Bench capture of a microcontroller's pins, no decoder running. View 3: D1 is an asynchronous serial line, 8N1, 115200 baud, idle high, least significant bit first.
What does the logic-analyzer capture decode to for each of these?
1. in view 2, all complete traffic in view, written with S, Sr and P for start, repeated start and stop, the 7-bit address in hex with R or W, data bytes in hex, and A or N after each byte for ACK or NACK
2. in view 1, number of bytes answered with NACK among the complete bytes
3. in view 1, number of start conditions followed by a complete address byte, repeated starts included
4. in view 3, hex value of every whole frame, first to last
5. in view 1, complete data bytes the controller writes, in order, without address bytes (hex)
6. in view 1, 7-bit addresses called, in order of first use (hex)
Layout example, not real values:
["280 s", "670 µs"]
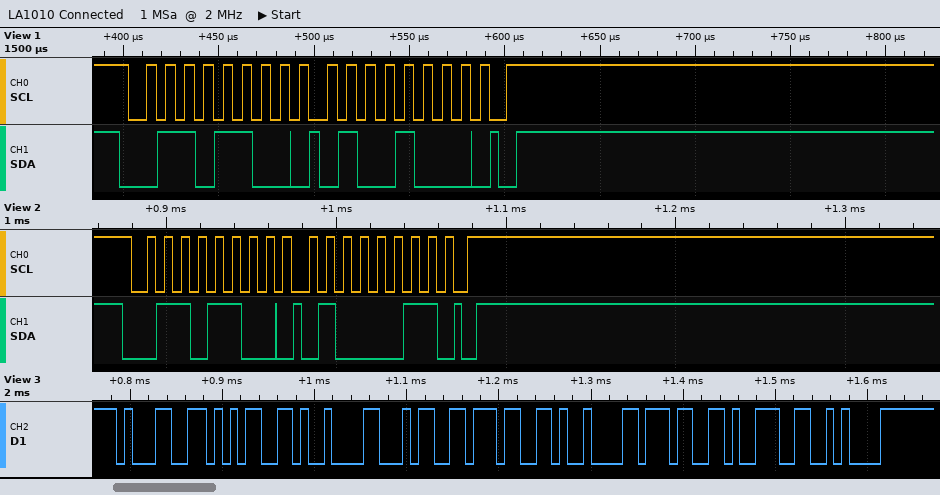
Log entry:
["S 36W A 43 A P", "0", "1", "31 35 09 34 37 09 37 39 0A", "48", "0x36"]
